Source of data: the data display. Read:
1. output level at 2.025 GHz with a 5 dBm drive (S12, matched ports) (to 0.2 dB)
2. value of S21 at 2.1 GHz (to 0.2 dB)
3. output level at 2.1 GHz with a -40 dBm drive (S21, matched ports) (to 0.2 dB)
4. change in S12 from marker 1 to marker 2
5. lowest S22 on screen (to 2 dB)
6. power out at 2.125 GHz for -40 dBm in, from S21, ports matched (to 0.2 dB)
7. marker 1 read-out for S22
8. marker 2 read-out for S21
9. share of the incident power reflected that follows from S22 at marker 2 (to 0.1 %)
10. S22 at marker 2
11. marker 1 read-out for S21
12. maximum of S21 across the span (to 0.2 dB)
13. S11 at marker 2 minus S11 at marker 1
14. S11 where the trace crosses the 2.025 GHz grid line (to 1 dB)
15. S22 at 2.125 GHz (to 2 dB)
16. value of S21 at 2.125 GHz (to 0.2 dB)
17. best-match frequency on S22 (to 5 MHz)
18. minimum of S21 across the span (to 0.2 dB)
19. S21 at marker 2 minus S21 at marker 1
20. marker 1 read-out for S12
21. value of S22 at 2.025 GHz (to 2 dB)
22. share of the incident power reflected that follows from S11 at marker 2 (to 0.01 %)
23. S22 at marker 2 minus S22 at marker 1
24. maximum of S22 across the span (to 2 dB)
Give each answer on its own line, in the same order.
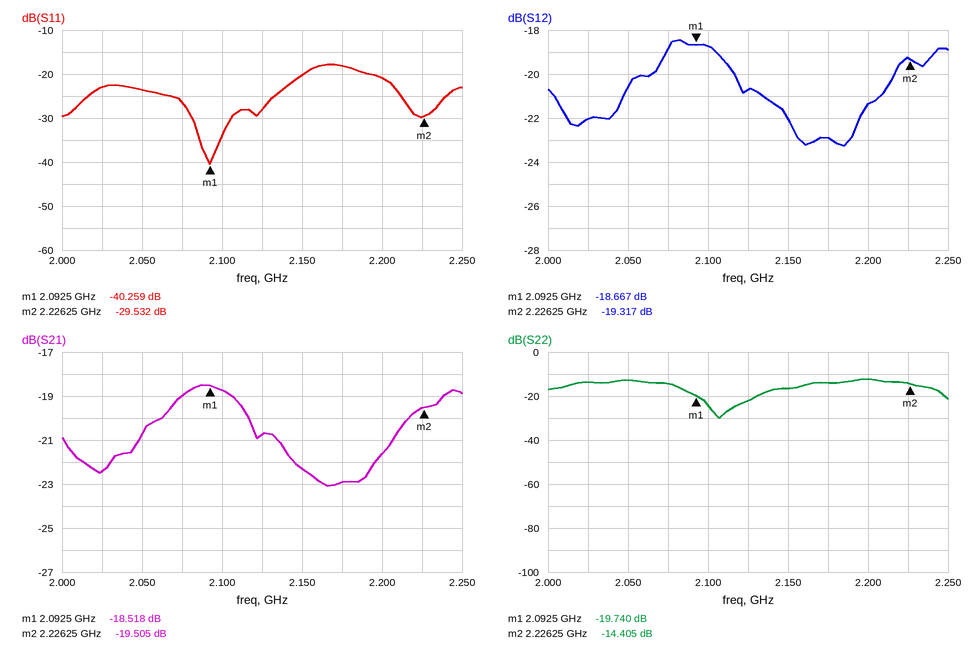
-17.0 dBm
-18.8 dB
-58.8 dBm
-0.650 dB
-30 dB
-60.8 dBm
-19.740 dB
-19.505 dB
3.6 %
-14.405 dB
-18.518 dB
-18.4 dB
10.727 dB
-23 dB
-22 dB
-20.8 dB
2.105 GHz
-23.0 dB
-0.987 dB
-18.667 dB
-14 dB
0.11 %
5.335 dB
-12 dB
